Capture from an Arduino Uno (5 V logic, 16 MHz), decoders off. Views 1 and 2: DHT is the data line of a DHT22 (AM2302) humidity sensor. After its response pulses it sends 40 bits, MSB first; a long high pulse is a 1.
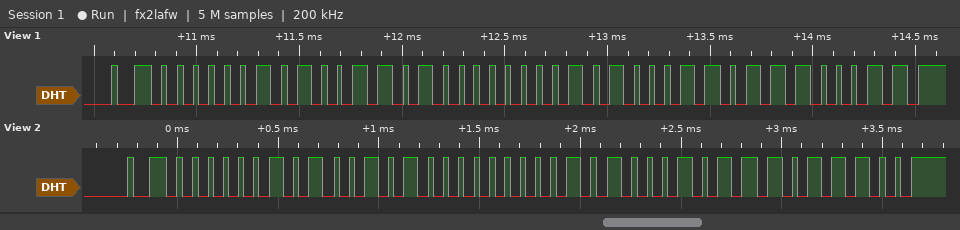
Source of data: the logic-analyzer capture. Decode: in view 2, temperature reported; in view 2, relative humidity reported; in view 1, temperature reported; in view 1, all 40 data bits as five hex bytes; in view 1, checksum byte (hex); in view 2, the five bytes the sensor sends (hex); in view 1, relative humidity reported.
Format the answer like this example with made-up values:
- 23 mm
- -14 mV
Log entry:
- 32.5 °C
- 66.0 %
- 32.6 °C
- 02 9A 01 46 E3
- 0xE3
- 02 94 01 45 DC
- 66.6 %
